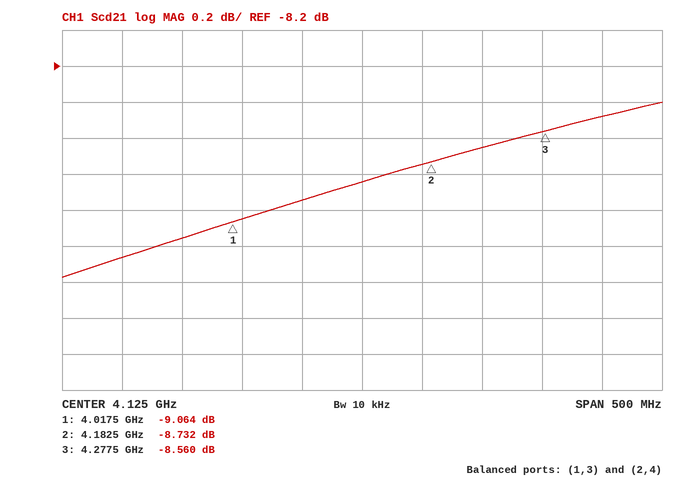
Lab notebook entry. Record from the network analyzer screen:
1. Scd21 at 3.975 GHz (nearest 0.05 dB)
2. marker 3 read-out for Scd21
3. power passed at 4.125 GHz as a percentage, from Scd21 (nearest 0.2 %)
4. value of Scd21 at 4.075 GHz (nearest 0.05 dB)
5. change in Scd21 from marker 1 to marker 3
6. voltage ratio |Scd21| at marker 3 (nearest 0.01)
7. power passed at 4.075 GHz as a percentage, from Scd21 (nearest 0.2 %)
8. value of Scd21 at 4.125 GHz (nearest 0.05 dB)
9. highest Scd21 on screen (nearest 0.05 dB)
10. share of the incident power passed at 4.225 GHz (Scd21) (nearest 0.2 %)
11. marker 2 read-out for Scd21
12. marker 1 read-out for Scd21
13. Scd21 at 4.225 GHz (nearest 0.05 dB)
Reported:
-9.15 dB
-8.560 dB
13.0 %
-8.95 dB
0.504 dB
0.37
12.8 %
-8.85 dB
-8.40 dB
13.6 %
-8.732 dB
-9.064 dB
-8.65 dB
